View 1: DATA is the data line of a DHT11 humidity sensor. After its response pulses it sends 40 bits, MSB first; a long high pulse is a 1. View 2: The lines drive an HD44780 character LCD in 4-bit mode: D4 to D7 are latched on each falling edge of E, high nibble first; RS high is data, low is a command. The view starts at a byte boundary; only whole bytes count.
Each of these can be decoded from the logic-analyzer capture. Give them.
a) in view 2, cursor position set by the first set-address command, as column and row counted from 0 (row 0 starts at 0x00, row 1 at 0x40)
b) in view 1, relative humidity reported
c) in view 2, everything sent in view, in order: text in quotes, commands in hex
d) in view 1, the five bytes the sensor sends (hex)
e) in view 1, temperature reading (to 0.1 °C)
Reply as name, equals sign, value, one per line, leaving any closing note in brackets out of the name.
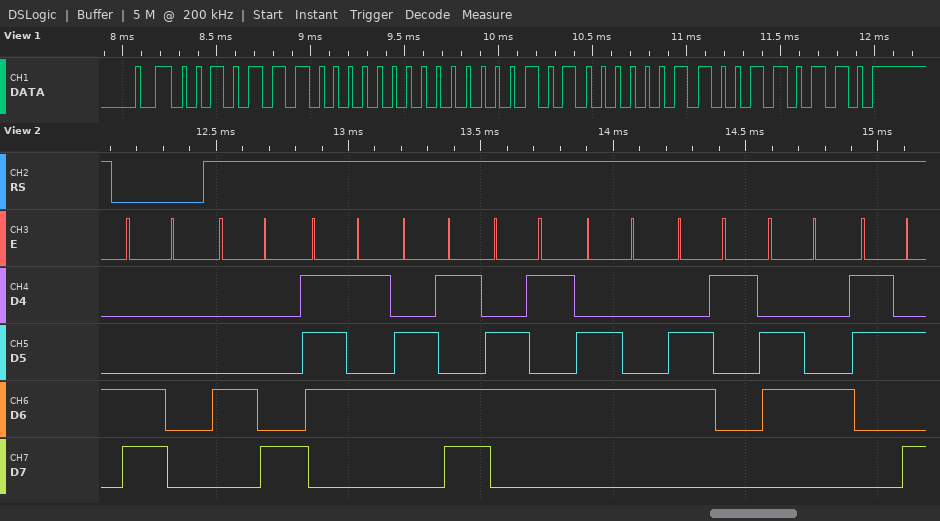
in view 2, cursor position set by the first set-address command, as column and row counted from 0 = column 0, row 1
in view 1, relative humidity reported = 46 %
in view 2, everything sent in view, in order: text in quotes, commands in hex = 0xC0 "Humedad:"
in view 1, the five bytes the sensor sends = 2E 00 05 03 36
in view 1, temperature reading = 5.3 °C
